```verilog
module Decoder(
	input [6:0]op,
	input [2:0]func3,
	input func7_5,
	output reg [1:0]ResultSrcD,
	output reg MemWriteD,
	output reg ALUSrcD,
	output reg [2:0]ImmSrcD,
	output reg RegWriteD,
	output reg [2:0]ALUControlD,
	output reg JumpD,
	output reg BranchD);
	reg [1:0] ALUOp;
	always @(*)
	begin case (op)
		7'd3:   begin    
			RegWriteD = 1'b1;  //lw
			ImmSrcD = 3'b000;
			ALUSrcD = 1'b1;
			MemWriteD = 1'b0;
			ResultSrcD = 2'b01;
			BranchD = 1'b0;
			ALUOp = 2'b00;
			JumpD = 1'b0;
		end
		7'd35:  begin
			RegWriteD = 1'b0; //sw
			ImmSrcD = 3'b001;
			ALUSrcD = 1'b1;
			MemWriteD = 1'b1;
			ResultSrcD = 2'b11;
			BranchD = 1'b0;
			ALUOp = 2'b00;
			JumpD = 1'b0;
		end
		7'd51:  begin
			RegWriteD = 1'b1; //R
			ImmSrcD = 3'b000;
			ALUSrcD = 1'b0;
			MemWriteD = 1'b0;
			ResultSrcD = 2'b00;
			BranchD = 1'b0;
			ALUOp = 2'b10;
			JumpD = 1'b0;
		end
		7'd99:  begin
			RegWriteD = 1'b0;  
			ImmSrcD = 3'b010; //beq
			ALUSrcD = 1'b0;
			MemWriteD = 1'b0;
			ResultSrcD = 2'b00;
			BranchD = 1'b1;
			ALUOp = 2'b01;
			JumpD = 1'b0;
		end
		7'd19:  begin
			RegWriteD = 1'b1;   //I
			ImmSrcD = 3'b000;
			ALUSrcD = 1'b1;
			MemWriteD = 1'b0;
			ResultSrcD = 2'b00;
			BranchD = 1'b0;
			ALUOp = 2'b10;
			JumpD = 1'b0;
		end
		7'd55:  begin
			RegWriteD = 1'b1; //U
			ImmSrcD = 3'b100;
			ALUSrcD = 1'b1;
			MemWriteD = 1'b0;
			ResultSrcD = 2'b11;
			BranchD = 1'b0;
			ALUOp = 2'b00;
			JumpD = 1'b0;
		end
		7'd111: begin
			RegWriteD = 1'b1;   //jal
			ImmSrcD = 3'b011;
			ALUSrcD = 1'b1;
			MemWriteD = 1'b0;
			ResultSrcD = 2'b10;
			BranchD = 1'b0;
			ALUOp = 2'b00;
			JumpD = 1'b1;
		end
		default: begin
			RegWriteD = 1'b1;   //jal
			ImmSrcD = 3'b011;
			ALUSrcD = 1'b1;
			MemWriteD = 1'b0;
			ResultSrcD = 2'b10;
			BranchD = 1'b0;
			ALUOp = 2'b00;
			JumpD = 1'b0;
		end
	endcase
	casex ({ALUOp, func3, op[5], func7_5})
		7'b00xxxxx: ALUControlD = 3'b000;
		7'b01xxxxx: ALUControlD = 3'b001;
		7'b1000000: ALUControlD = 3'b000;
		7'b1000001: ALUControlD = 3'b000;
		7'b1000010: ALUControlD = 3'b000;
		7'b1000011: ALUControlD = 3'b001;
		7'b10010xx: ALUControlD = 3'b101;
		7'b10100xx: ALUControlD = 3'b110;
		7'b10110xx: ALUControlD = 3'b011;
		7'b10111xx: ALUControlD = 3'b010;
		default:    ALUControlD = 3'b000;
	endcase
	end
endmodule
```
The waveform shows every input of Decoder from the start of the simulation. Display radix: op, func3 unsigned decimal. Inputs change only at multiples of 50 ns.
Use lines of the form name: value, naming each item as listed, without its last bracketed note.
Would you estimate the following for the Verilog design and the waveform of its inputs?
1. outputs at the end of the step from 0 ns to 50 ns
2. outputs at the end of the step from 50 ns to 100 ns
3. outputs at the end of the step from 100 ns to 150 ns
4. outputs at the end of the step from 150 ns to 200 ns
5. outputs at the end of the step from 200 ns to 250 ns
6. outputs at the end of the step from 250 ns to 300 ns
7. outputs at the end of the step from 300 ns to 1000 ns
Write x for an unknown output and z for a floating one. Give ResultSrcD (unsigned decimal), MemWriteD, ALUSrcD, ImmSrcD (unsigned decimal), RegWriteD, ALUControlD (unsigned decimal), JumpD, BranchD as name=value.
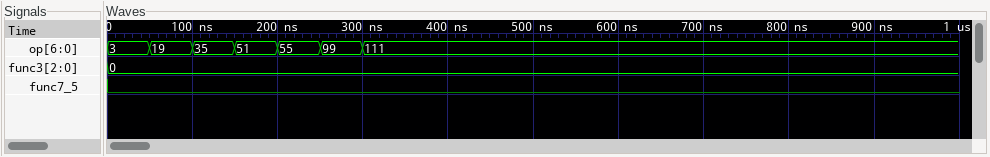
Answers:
outputs at the end of the step from 0 ns to 50 ns: ResultSrcD=1, MemWriteD=0, ALUSrcD=1, ImmSrcD=0, RegWriteD=1, ALUControlD=0, JumpD=0, BranchD=0
outputs at the end of the step from 50 ns to 100 ns: ResultSrcD=0, MemWriteD=0, ALUSrcD=1, ImmSrcD=0, RegWriteD=1, ALUControlD=0, JumpD=0, BranchD=0
outputs at the end of the step from 100 ns to 150 ns: ResultSrcD=3, MemWriteD=1, ALUSrcD=1, ImmSrcD=1, RegWriteD=0, ALUControlD=0, JumpD=0, BranchD=0
outputs at the end of the step from 150 ns to 200 ns: ResultSrcD=0, MemWriteD=0, ALUSrcD=0, ImmSrcD=0, RegWriteD=1, ALUControlD=0, JumpD=0, BranchD=0
outputs at the end of the step from 200 ns to 250 ns: ResultSrcD=3, MemWriteD=0, ALUSrcD=1, ImmSrcD=4, RegWriteD=1, ALUControlD=0, JumpD=0, BranchD=0
outputs at the end of the step from 250 ns to 300 ns: ResultSrcD=0, MemWriteD=0, ALUSrcD=0, ImmSrcD=2, RegWriteD=0, ALUControlD=1, JumpD=0, BranchD=1
outputs at the end of the step from 300 ns to 1000 ns: ResultSrcD=2, MemWriteD=0, ALUSrcD=1, ImmSrcD=3, RegWriteD=1, ALUControlD=0, JumpD=1, BranchD=0
